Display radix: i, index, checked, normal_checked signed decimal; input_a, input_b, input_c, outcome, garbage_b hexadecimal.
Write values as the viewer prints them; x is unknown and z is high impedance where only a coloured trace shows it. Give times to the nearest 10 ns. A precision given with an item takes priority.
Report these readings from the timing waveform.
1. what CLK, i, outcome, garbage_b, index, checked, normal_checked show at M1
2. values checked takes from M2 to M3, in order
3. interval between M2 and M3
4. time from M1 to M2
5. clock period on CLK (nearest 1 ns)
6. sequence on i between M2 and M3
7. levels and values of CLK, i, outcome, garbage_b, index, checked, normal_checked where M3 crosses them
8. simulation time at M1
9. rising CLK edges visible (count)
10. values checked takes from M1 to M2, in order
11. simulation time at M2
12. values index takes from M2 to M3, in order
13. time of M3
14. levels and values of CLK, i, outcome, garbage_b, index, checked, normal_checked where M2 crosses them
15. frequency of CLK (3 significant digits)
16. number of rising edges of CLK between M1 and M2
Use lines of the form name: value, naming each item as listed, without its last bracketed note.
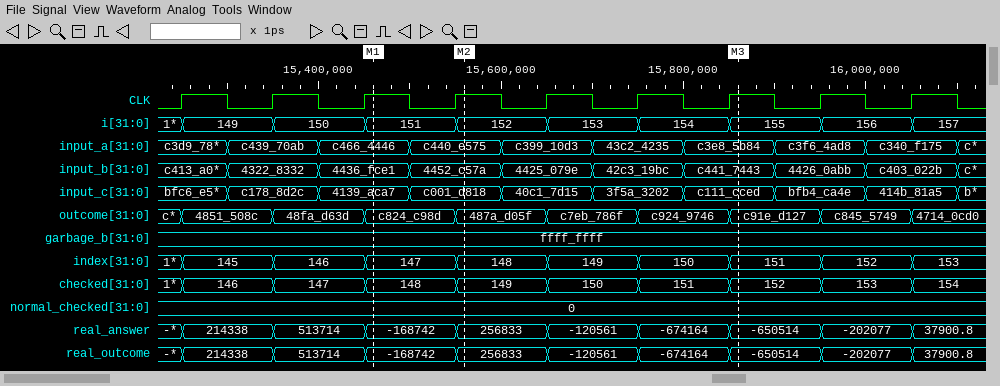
what CLK, i, outcome, garbage_b, index, checked, normal_checked show at M1: CLK=1, i=151, outcome=c824_c98d, garbage_b=ffff_ffff, index=147, checked=148, normal_checked=0
values checked takes from M2 to M3, in order: 149, 150, 151, 152
interval between M2 and M3: 300 ns
time from M1 to M2: 100 ns
clock period on CLK: 100 ns
sequence on i between M2 and M3: 152, 153, 154, 155
levels and values of CLK, i, outcome, garbage_b, index, checked, normal_checked where M3 crosses them: CLK=1, i=155, outcome=c91e_d127, garbage_b=ffff_ffff, index=151, checked=152, normal_checked=0
simulation time at M1: 15460 ns
rising CLK edges visible: 9
values checked takes from M1 to M2, in order: 148, 149
simulation time at M2: 15560 ns
values index takes from M2 to M3, in order: 148, 149, 150, 151
time of M3: 15860 ns
levels and values of CLK, i, outcome, garbage_b, index, checked, normal_checked where M2 crosses them: CLK=1, i=152, outcome=487a_d05f, garbage_b=ffff_ffff, index=148, checked=149, normal_checked=0
frequency of CLK: 10.0 MHz
number of rising edges of CLK between M1 and M2: 1
